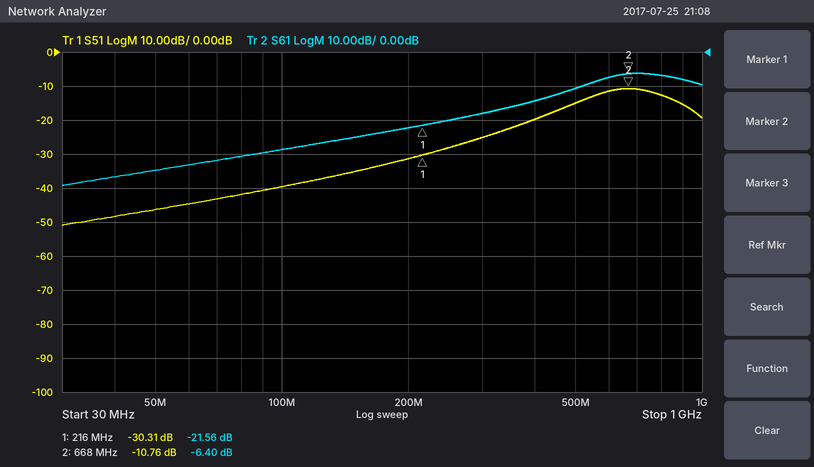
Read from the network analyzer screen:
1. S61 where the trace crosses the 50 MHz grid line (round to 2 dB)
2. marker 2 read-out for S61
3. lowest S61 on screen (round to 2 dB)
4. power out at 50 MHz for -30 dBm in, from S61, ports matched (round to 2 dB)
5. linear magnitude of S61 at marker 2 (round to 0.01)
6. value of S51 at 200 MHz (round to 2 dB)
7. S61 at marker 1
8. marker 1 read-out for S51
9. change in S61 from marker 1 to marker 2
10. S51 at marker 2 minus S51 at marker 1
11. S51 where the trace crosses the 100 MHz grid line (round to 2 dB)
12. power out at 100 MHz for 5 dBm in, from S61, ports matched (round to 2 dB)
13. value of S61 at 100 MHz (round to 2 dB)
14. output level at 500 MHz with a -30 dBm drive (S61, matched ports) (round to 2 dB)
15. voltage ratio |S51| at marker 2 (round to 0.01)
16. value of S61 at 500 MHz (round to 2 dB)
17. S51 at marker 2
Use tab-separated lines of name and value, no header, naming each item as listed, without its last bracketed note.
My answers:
S61 where the trace crosses the 50 MHz grid line	-34 dB
marker 2 read-out for S61	-6.40 dB
lowest S61 on screen	-40 dB
power out at 50 MHz for -30 dBm in, from S61, ports matched	-64 dBm
linear magnitude of S61 at marker 2	0.48
value of S51 at 200 MHz	-32 dB
S61 at marker 1	-21.56 dB
marker 1 read-out for S51	-30.31 dB
change in S61 from marker 1 to marker 2	15.16 dB
S51 at marker 2 minus S51 at marker 1	19.55 dB
S51 where the trace crosses the 100 MHz grid line	-40 dB
power out at 100 MHz for 5 dBm in, from S61, ports matched	-24 dBm
value of S61 at 100 MHz	-28 dB
output level at 500 MHz with a -30 dBm drive (S61, matched ports)	-40 dBm
voltage ratio |S51| at marker 2	0.29
value of S61 at 500 MHz	-10 dB
S51 at marker 2	-10.76 dB
